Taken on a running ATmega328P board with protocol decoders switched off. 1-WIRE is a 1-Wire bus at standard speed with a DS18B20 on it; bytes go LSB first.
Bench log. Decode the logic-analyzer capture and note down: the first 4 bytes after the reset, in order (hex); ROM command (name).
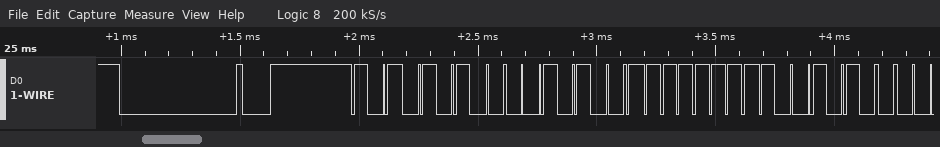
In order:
55 28 FF 29
Match ROM
